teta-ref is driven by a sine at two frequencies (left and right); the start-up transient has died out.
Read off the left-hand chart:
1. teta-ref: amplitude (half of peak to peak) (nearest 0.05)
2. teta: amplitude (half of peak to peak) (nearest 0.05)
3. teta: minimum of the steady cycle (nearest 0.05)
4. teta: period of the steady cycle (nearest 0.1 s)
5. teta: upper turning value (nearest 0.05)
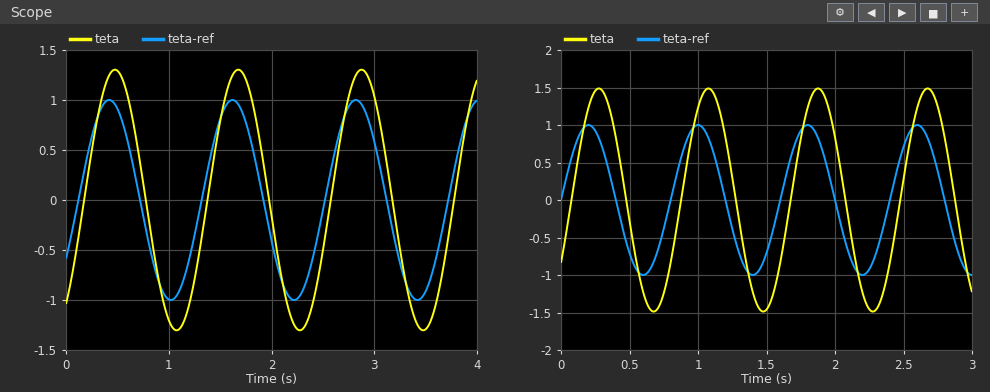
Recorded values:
1.00
1.30
-1.30
1.2 s
1.30
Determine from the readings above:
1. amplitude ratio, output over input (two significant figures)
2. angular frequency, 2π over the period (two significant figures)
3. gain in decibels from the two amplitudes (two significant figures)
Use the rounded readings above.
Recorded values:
1.3
5.2 rad/s
2.3 dB
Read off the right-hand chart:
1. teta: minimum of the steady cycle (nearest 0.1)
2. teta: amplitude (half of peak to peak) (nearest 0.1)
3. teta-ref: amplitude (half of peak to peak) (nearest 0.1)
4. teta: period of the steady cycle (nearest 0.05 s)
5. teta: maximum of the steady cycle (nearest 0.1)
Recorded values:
-1.5
1.5
1.0
0.80 s
1.5
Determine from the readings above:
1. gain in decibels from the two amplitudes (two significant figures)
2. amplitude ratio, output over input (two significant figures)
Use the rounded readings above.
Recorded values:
3.5 dB
1.5
